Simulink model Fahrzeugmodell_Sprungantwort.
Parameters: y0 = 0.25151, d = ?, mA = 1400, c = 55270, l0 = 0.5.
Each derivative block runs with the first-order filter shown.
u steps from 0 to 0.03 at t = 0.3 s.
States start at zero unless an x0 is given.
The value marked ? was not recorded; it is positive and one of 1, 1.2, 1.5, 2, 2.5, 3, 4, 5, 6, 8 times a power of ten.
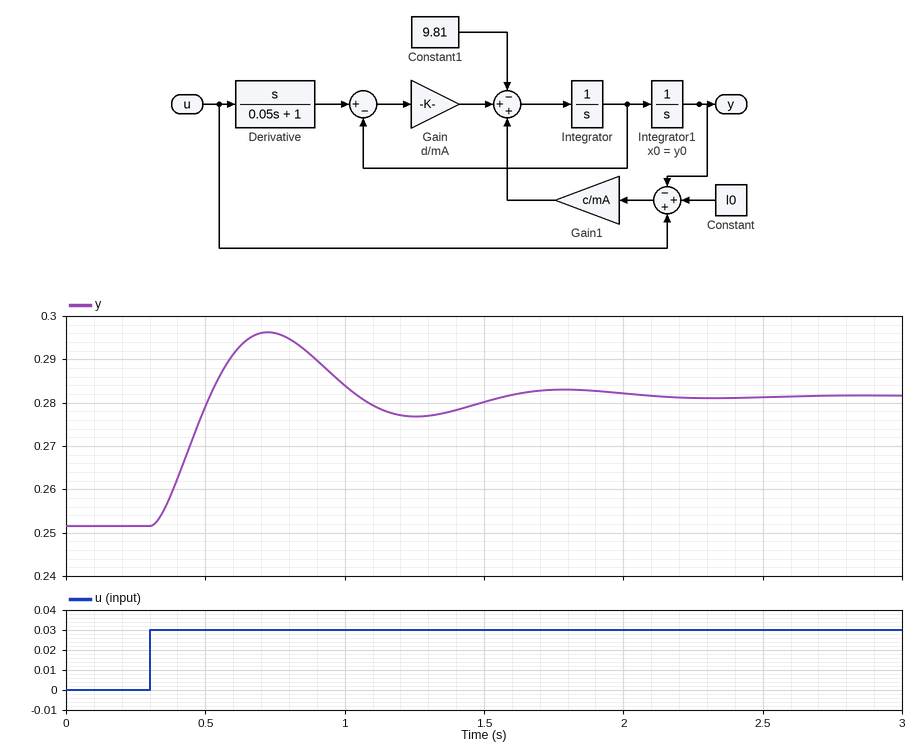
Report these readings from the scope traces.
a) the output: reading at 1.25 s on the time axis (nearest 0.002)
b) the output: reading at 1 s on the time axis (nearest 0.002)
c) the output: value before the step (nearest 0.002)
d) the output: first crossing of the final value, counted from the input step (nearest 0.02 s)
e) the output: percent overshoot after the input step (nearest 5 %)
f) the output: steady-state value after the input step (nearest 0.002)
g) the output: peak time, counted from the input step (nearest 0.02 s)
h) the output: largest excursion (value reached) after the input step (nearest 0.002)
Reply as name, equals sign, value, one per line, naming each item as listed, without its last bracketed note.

the output: reading at 1.25 s on the time axis = 0.276
the output: reading at 1 s on the time axis = 0.284
the output: value before the step = 0.252
the output: first crossing of the final value, counted from the input step = 0.22 s
the output: percent overshoot after the input step = 50 %
the output: steady-state value after the input step = 0.282
the output: peak time, counted from the input step = 0.42 s
the output: largest excursion (value reached) after the input step = 0.296
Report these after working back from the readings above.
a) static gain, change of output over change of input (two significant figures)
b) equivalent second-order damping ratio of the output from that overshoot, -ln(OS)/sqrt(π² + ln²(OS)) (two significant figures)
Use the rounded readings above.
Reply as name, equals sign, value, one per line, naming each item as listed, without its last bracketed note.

static gain, change of output over change of input = 1.0
equivalent second-order damping ratio of the output from that overshoot, -ln(OS)/sqrt(π² + ln²(OS)) = 0.22
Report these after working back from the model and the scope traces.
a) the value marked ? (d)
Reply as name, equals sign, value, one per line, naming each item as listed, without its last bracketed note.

the value marked ? = 6000
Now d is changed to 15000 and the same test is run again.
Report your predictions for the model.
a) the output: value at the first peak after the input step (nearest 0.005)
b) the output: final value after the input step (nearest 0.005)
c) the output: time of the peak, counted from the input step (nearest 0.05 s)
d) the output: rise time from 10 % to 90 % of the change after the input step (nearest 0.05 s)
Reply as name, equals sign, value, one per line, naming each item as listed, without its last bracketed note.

the output: value at the first peak after the input step = 0.290
the output: final value after the input step = 0.280
the output: time of the peak, counted from the input step = 0.35 s
the output: rise time from 10 % to 90 % of the change after the input step = 0.15 s
